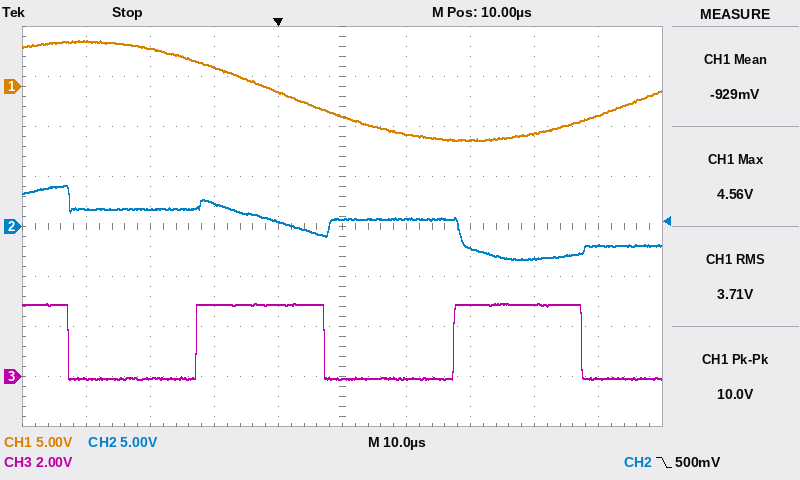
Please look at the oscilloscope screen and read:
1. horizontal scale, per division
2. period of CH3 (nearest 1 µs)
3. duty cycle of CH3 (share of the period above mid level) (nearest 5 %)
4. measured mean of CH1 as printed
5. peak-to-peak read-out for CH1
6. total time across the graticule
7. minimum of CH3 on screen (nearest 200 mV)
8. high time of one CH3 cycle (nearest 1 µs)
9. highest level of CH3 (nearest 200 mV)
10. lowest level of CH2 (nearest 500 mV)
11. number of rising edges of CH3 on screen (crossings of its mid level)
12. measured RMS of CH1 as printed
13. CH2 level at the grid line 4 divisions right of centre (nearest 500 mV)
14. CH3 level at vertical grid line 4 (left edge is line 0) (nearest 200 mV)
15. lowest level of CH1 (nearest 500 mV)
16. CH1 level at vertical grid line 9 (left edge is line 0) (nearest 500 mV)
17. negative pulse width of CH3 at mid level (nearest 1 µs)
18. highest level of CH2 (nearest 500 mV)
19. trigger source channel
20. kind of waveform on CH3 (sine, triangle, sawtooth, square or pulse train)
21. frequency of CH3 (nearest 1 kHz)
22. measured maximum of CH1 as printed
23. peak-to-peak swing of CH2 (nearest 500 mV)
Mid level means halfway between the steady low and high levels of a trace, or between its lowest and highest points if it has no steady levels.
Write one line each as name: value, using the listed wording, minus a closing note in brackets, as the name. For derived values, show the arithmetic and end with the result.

horizontal scale, per division: 10 µs
period of CH3: 40 µs
duty cycle of CH3 (share of the period above mid level): 20 µs / 40 µs ≈ 50 %
measured mean of CH1 as printed: -929 mV
peak-to-peak read-out for CH1: 10.0 V
total time across the graticule: 100 µs
minimum of CH3 on screen: -200 mV
high time of one CH3 cycle: 20 µs
highest level of CH3: 3.0 V
lowest level of CH2: -3.5 V
number of rising edges of CH3 on screen: 2
measured RMS of CH1 as printed: 3.71 V
CH2 level at the grid line 4 divisions right of centre: -2.0 V
CH3 level at vertical grid line 4 (left edge is line 0): 2.8 V
lowest level of CH1: -5.5 V
CH1 level at vertical grid line 9 (left edge is line 0): -3.0 V
negative pulse width of CH3 at mid level: 20 µs
highest level of CH2: 4.0 V
trigger source channel: CH2
kind of waveform on CH3: square
frequency of CH3: 1 / 40 µs ≈ 25 kHz
measured maximum of CH1 as printed: 4.56 V
peak-to-peak swing of CH2: 4.0 V − (-3.5 V) = 7.5 V
